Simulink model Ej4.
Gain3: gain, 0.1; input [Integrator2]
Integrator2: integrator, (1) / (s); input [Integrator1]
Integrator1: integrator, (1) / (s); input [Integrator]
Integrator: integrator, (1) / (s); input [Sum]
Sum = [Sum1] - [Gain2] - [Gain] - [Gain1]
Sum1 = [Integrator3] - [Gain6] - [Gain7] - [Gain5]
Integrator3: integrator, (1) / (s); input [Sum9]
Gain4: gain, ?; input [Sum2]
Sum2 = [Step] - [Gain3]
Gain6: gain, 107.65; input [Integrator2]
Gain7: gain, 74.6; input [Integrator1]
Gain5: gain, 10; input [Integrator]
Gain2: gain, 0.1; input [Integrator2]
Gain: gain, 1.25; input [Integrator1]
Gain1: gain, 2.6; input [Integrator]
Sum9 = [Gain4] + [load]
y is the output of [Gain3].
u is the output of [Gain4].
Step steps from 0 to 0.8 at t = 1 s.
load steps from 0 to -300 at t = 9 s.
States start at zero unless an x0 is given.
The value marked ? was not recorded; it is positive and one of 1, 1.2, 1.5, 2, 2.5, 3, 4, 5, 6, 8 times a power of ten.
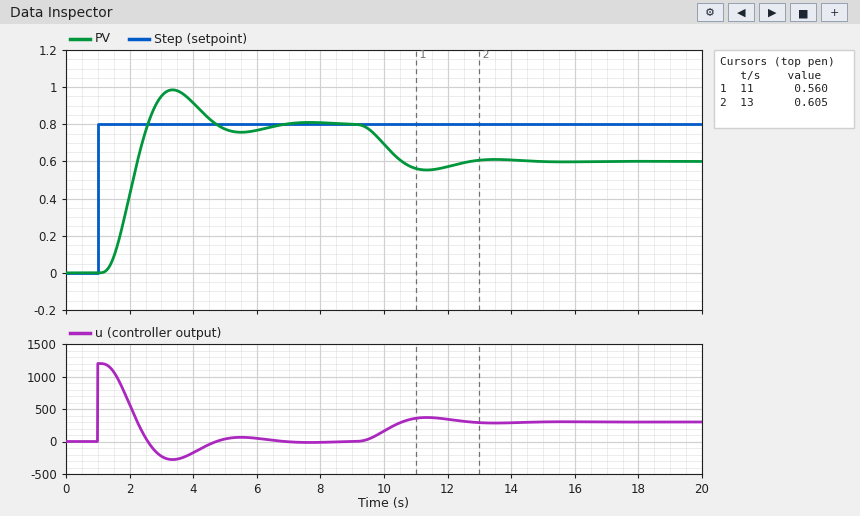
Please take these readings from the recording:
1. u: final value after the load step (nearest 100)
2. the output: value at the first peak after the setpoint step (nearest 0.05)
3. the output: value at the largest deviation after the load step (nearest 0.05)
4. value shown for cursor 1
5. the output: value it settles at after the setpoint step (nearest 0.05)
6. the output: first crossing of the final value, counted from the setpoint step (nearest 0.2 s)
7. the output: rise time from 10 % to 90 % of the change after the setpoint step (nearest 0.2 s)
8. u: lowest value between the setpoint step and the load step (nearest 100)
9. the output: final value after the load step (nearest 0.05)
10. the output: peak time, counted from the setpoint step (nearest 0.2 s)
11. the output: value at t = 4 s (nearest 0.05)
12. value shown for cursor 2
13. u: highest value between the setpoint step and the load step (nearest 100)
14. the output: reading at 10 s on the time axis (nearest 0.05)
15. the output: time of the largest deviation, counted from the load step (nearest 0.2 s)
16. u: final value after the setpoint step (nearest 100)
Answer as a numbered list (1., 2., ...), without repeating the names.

1. 300
2. 1.00
3. 0.55
4. 0.560
5. 0.80
6. 1.6 s
7. 1.0 s
8. -300
9. 0.60
10. 2.4 s
11. 0.90
12. 0.605
13. 1200
14. 0.70
15. 2.4 s
16. 0
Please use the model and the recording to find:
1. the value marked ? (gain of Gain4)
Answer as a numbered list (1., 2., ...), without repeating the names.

1. 1500
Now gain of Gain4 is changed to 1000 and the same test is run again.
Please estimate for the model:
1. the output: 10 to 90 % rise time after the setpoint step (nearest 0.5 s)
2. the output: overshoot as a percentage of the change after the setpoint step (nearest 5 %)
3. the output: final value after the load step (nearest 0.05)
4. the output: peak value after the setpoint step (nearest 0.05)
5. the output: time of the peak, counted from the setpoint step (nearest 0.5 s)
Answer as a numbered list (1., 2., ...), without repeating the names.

1. 1.5 s
2. 10 %
3. 0.50
4. 0.90
5. 3.0 s
